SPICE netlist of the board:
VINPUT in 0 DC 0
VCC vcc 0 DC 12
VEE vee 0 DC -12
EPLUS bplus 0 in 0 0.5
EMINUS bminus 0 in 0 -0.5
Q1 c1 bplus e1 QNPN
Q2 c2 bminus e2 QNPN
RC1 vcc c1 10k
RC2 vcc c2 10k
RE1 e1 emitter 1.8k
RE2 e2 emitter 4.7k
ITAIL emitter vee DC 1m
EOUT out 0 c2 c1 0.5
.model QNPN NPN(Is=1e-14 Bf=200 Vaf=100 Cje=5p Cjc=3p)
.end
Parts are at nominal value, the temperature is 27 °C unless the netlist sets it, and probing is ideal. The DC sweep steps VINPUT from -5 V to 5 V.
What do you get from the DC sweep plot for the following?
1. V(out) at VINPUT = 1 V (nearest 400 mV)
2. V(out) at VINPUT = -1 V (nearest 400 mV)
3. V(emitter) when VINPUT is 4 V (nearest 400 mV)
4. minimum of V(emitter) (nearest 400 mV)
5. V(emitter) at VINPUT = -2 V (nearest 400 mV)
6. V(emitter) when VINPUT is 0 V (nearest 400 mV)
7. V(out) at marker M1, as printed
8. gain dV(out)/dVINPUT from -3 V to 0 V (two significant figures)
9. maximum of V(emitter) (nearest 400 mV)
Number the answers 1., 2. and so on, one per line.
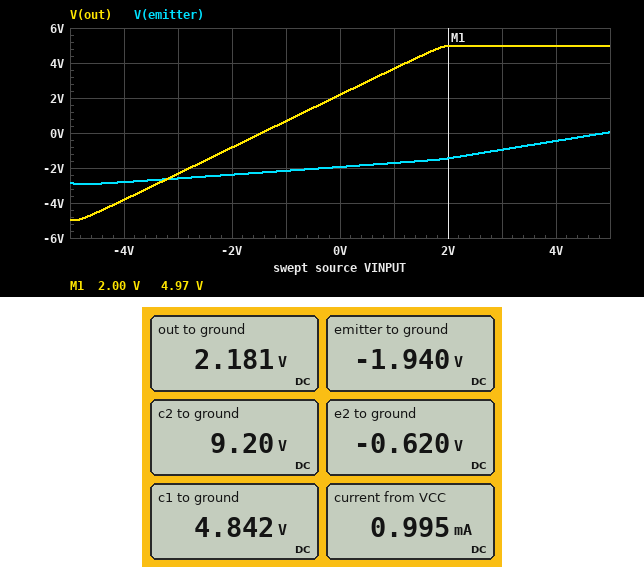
1. 3.6 V
2. 800 mV
3. -400 mV
4. -2.8 V
5. -2.4 V
6. -2.0 V
7. 4.97 V
8. 1.5 V/V
9. 0 V
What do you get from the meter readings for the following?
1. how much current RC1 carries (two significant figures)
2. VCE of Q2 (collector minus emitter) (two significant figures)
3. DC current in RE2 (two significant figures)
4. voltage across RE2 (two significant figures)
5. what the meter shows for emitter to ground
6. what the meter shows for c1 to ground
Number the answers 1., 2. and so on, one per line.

1. 720 µA
2. 9.8 V
3. 280 µA
4. 1.3 V
5. -1.940 V
6. 4.842 V
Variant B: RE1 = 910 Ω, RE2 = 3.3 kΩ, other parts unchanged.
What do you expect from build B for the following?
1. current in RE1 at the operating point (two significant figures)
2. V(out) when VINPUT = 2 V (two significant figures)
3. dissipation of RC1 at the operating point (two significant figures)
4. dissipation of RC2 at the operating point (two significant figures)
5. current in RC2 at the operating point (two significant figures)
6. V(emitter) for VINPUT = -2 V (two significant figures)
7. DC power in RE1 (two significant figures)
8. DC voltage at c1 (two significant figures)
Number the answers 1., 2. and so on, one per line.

1. 780 µA
2. 5.0 V
3. 6.0 mW
4. 500 µW
5. 220 µA
6. -1.9 V
7. 550 µW
8. 4.3 V
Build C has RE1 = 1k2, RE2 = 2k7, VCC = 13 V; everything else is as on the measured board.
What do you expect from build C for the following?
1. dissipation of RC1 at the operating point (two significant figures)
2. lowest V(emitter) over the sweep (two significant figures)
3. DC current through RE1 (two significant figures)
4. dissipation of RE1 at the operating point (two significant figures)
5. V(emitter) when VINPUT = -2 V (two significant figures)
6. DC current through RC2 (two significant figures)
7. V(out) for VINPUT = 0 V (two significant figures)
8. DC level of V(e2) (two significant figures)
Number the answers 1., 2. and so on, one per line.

1. 4.7 mW
2. -1.9 V
3. 690 µA
4. 570 µW
5. -1.8 V
6. 310 µA
7. 1.9 V
8. -620 mV
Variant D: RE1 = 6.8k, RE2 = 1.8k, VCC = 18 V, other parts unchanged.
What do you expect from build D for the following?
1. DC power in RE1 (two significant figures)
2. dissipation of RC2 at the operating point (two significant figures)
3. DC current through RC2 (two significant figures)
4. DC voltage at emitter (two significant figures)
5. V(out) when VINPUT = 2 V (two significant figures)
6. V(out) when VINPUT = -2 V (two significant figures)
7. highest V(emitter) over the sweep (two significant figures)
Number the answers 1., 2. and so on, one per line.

1. 310 µW
2. 6.1 mW
3. 780 µA
4. -2.1 V
5. -570 mV
6. -5.0 V
7. 46 mV
